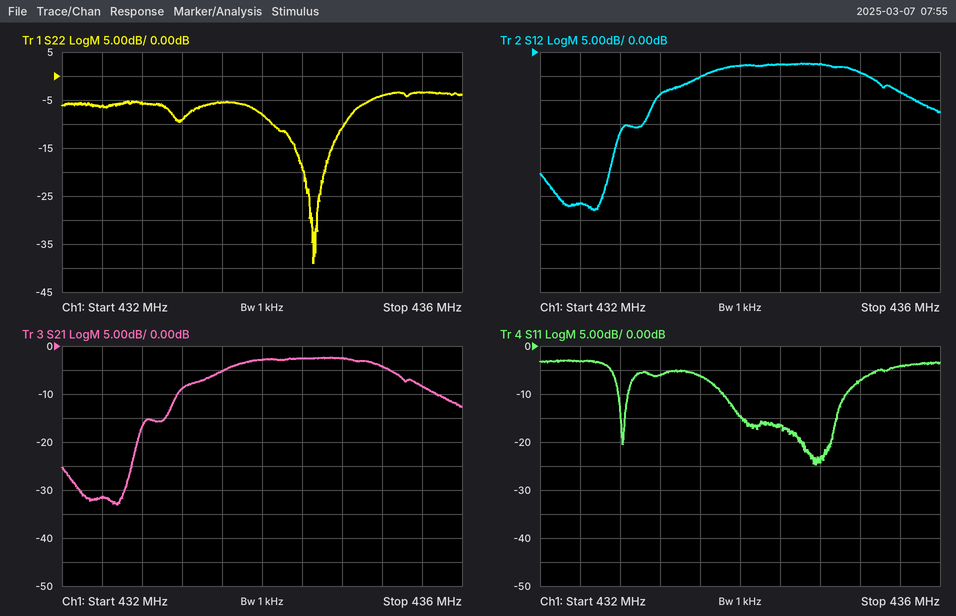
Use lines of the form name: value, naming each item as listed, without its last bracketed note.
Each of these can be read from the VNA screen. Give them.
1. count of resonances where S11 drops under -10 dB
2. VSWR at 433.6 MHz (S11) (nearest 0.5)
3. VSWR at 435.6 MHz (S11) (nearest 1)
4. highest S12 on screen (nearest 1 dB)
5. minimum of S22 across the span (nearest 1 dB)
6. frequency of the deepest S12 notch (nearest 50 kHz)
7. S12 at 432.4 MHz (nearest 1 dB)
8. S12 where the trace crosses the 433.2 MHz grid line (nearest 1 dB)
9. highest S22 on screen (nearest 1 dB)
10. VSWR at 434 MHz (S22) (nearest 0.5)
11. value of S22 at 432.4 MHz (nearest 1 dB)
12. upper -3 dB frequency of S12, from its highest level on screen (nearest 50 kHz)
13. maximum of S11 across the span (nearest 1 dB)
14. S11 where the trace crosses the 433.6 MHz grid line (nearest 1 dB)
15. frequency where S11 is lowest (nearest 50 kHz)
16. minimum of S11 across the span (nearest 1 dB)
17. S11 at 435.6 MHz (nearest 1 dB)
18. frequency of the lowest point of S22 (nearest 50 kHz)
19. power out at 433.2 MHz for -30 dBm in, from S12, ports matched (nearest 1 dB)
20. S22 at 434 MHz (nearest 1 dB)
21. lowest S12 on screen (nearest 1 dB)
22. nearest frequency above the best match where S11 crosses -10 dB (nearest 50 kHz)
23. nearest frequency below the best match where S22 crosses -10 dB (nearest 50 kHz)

count of resonances where S11 drops under -10 dB: 2
VSWR at 433.6 MHz (S11): 3.0
VSWR at 435.6 MHz (S11): 4
highest S12 on screen: -2 dB
minimum of S22 across the span: -39 dB
frequency of the deepest S12 notch: 432.55 MHz
S12 at 432.4 MHz: -32 dB
S12 where the trace crosses the 433.2 MHz grid line: -9 dB
highest S22 on screen: -3 dB
VSWR at 434 MHz (S22): 2.5
value of S22 at 432.4 MHz: -6 dB
upper -3 dB frequency of S12, from its highest level on screen: 435.30 MHz
maximum of S11 across the span: -3 dB
S11 where the trace crosses the 433.6 MHz grid line: -6 dB
frequency where S11 is lowest: 434.75 MHz
minimum of S11 across the span: -25 dB
S11 at 435.6 MHz: -4 dB
frequency of the lowest point of S22: 434.50 MHz
power out at 433.2 MHz for -30 dBm in, from S12, ports matched: -39 dBm
S22 at 434 MHz: -8 dB
lowest S12 on screen: -33 dB
nearest frequency above the best match where S11 crosses -10 dB: 435.05 MHz
nearest frequency below the best match where S22 crosses -10 dB: 434.10 MHz
